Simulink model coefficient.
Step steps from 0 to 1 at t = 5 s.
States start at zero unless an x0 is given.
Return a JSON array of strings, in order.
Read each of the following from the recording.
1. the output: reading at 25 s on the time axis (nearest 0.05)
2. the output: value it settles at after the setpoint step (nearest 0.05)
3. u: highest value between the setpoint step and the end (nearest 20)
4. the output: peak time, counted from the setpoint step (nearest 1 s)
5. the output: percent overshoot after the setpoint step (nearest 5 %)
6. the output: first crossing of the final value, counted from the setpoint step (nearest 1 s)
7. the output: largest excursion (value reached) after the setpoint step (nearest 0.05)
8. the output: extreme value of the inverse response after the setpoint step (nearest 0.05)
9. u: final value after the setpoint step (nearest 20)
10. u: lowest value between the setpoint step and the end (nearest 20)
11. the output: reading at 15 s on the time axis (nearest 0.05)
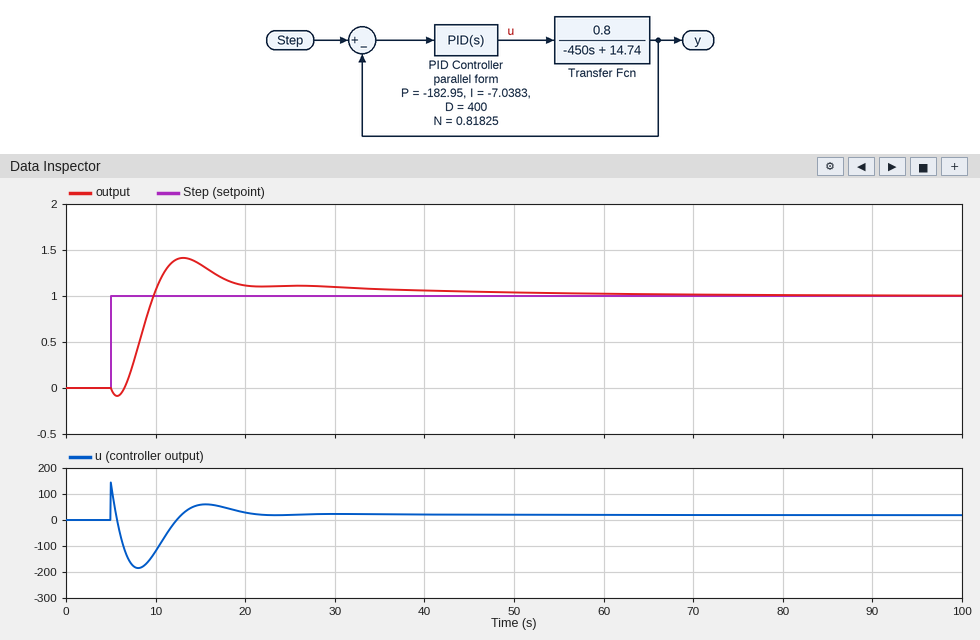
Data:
["1.10", "1.00", "140", "8 s", "40 %", "5 s", "1.40", "-0.10", "20", "-180", "1.35"]
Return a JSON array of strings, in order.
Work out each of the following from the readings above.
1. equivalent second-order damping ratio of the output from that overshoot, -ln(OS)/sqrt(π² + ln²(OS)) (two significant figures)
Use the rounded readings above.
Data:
["0.28"]
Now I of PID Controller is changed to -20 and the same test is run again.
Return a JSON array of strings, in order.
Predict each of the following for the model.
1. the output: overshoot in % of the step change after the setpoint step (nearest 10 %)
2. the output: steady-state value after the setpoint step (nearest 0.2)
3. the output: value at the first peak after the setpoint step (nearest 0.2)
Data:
["60 %", "1.0", "1.6"]
